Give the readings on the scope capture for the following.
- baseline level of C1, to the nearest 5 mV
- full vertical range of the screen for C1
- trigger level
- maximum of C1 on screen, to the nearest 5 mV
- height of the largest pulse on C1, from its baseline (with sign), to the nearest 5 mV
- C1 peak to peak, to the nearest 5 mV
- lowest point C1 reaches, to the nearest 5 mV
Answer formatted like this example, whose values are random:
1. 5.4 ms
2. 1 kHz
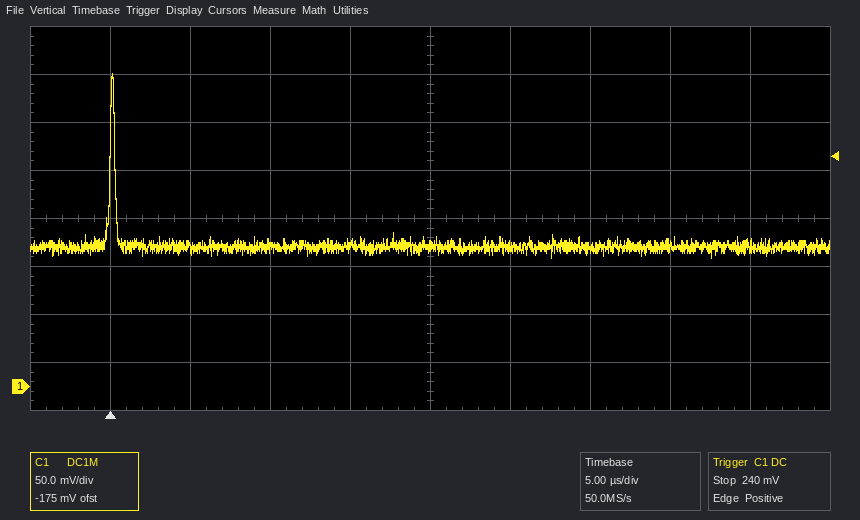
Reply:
1. 145 mV
2. 400 mV
3. 240 mV
4. 325 mV
5. +180 mV
6. 190 mV
7. 135 mV
